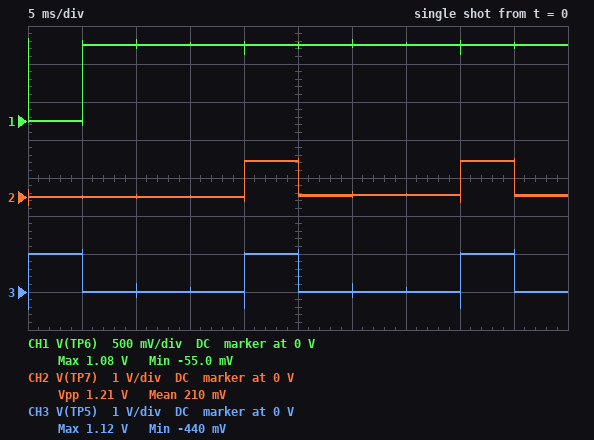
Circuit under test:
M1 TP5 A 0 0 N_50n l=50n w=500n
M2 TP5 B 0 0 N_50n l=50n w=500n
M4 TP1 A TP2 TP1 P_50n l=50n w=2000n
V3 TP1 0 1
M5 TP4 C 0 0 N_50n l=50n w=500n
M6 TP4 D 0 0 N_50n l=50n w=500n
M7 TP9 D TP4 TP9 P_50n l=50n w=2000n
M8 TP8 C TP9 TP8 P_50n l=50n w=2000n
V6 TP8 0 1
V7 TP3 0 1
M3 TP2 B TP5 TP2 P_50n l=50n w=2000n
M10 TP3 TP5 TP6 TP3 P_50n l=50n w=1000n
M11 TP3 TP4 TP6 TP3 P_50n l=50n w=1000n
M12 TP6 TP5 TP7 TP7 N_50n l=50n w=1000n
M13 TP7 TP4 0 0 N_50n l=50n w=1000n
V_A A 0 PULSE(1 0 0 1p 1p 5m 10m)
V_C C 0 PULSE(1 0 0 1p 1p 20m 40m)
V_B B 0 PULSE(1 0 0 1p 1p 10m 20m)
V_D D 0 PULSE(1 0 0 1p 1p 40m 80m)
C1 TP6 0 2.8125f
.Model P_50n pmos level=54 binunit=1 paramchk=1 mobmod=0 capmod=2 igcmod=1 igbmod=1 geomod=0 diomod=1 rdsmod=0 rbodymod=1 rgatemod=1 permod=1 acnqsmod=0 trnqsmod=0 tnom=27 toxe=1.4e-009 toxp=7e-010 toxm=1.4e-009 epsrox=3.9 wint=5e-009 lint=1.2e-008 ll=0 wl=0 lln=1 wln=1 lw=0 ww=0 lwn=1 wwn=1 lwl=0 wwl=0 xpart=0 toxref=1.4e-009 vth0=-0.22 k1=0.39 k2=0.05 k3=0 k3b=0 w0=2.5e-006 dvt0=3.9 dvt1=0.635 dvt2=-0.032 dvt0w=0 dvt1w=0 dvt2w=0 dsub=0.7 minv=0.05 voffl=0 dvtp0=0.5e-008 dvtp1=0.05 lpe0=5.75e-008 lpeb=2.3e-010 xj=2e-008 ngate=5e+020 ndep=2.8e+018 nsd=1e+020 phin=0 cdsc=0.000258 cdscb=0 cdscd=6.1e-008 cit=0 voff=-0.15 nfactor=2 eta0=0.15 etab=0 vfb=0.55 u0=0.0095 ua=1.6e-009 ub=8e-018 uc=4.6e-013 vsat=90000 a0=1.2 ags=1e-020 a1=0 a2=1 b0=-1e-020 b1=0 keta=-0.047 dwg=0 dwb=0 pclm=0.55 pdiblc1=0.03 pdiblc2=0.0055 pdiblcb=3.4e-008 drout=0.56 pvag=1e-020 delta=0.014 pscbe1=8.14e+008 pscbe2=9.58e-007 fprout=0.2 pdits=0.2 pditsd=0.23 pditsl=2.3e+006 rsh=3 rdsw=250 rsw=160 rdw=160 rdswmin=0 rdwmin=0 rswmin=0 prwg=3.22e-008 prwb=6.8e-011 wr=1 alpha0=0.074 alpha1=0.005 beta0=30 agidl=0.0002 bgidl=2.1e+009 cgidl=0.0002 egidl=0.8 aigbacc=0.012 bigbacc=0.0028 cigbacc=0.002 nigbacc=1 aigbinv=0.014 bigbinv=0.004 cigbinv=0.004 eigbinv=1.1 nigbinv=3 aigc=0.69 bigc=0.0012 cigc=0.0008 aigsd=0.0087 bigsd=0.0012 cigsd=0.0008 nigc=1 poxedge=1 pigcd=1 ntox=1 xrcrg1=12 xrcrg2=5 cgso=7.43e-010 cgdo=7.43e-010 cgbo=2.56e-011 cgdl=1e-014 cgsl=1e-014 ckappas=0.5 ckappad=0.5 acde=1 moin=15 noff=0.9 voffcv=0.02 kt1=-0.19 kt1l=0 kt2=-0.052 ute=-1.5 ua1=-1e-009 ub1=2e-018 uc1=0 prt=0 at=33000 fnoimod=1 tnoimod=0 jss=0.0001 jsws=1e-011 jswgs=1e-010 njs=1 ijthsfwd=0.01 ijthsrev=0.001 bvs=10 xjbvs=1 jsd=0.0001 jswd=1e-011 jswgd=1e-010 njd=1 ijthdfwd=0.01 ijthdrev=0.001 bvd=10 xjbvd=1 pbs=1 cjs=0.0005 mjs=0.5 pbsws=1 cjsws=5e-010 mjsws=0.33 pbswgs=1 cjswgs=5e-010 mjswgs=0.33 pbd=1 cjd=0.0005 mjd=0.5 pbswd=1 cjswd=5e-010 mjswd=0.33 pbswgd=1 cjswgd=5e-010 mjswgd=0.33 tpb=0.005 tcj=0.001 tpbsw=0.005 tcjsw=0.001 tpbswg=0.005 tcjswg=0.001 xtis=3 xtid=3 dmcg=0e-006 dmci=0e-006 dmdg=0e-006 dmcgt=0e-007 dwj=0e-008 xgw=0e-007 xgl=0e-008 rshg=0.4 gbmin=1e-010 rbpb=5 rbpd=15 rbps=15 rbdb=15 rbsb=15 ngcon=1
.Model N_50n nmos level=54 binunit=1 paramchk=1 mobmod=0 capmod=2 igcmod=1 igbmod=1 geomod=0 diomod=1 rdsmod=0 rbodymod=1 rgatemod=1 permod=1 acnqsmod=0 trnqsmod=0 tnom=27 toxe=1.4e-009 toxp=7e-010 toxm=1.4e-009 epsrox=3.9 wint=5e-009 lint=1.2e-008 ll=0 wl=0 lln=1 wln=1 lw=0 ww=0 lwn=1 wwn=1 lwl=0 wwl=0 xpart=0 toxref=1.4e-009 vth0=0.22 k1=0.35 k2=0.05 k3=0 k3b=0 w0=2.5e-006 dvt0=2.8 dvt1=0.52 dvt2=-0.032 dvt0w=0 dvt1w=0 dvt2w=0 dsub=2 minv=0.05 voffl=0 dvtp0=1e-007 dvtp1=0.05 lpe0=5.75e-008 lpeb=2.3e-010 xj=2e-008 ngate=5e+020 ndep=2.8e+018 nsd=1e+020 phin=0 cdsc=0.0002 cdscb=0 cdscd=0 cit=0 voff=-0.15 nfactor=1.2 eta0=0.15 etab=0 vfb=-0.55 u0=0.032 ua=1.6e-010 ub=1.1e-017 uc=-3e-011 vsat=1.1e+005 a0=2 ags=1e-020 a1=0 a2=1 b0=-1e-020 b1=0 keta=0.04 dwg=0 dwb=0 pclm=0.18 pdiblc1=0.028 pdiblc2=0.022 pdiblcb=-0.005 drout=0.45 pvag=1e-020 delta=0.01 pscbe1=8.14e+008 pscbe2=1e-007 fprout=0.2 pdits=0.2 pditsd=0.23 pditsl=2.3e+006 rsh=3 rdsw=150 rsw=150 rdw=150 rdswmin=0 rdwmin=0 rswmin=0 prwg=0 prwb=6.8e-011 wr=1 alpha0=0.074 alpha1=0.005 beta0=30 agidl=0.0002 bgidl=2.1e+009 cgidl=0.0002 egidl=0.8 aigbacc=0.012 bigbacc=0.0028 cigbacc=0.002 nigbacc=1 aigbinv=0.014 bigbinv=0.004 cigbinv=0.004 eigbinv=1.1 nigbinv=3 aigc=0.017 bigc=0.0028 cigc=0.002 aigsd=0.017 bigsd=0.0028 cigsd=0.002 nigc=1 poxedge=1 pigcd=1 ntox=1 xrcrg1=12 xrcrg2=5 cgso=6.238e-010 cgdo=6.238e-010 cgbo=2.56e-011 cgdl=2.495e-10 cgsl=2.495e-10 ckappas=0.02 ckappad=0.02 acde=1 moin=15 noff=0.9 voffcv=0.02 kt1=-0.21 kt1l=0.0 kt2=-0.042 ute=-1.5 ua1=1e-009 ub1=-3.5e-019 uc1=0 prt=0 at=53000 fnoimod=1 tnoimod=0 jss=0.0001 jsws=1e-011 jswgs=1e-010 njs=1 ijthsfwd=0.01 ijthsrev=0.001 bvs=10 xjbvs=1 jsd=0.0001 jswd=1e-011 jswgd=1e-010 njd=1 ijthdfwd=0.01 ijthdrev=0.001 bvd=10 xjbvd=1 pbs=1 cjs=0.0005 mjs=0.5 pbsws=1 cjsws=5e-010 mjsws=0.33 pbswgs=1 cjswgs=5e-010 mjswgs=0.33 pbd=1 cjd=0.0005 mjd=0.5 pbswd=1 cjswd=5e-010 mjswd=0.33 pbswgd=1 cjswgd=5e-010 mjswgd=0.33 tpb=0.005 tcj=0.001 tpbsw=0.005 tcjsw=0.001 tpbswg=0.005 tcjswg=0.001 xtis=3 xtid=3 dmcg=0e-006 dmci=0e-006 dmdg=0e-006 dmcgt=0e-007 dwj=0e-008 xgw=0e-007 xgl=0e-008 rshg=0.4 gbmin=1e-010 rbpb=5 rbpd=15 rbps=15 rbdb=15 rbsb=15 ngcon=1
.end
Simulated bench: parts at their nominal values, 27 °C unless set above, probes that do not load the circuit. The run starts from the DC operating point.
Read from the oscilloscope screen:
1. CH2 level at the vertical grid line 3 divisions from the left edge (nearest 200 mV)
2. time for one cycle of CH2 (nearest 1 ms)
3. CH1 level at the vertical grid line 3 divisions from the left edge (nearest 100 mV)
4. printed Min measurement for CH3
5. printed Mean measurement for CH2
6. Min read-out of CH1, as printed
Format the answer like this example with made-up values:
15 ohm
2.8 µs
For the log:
0 V
20 ms
1.0 V
-440 mV
210 mV
-55.0 mV
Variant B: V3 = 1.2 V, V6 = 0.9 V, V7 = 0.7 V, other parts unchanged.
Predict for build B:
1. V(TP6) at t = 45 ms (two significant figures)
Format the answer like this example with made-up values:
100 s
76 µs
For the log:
700 mV
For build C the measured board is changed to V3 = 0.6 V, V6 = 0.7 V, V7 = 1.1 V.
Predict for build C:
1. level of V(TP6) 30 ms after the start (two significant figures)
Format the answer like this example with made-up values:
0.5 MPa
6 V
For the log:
1.1 V
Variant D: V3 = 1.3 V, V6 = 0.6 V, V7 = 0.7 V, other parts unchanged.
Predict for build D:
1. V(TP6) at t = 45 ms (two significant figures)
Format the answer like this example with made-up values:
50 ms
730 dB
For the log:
700 mV
